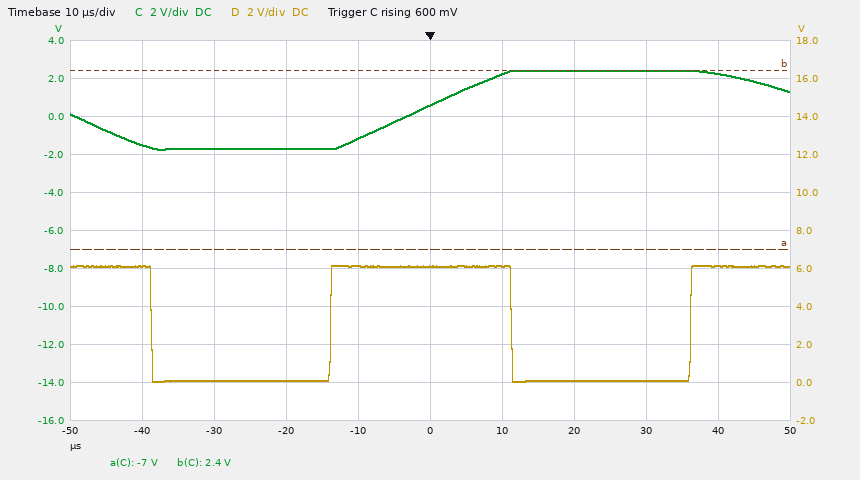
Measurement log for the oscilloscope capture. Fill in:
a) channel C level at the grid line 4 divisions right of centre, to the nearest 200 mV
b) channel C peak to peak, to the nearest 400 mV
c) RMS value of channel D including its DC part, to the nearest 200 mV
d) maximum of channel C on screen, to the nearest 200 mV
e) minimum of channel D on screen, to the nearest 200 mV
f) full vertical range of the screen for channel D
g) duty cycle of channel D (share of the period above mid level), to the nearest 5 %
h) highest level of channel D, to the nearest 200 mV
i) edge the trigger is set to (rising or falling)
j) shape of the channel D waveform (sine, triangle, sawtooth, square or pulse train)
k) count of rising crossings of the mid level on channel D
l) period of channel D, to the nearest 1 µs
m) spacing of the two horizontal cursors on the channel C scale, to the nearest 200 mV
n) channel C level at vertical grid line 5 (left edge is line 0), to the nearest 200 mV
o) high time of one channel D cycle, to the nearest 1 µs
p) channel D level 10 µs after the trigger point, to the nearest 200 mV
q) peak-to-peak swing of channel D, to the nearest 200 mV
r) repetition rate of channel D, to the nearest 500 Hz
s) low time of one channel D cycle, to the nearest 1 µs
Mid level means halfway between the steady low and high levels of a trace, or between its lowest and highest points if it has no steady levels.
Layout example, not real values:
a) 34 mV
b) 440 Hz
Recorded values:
a) 2.2 V
b) 4.0 V
c) 4.4 V
d) 2.4 V
e) 0.0 V
f) 20 V
g) 50 %
h) 6.2 V
i) rising
j) square
k) 2
l) 50 µs
m) 9.4 V
n) 600 mV
o) 25 µs
p) 6.2 V
q) 6.2 V
r) 20.0 kHz
s) 25 µs
